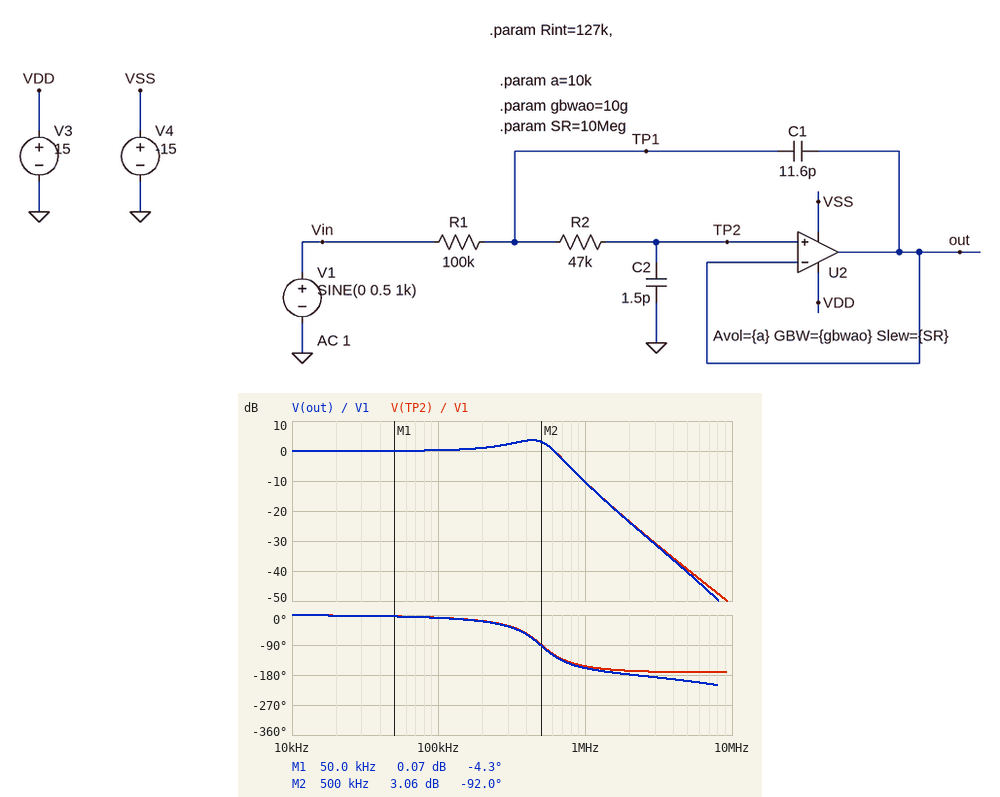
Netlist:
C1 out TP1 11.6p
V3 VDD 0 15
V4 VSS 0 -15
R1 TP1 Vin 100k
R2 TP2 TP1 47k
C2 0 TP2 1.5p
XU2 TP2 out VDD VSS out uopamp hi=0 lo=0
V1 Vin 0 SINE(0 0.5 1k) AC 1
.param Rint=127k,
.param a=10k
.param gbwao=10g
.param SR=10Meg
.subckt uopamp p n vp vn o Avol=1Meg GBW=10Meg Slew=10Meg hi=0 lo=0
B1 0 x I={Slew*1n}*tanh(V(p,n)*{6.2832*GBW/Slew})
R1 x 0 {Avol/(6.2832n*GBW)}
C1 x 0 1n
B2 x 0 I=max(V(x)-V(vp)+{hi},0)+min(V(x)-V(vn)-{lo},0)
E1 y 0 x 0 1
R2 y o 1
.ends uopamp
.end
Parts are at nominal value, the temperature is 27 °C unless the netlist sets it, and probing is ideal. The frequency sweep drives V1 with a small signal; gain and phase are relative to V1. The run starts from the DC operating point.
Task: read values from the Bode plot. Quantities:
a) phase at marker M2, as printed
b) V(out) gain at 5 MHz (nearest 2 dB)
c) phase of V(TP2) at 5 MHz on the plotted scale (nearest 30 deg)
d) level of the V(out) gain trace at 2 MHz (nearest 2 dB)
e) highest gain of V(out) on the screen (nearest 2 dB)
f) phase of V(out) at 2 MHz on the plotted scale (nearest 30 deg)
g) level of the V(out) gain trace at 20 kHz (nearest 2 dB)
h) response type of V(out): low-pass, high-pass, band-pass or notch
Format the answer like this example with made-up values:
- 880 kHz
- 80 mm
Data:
- -92.0 deg
- -40 dB
- -180 deg
- -24 dB
- 4 dB
- -180 deg
- 0 dB
- low-pass
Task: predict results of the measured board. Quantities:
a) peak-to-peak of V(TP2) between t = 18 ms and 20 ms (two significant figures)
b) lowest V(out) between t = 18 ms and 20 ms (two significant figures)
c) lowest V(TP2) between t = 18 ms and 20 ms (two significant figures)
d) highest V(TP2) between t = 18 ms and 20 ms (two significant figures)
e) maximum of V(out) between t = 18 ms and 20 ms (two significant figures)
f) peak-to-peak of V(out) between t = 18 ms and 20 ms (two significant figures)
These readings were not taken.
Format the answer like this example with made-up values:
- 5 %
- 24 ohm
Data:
- 1.0 V
- -500 mV
- -500 mV
- 500 mV
- 500 mV
- 1.0 V
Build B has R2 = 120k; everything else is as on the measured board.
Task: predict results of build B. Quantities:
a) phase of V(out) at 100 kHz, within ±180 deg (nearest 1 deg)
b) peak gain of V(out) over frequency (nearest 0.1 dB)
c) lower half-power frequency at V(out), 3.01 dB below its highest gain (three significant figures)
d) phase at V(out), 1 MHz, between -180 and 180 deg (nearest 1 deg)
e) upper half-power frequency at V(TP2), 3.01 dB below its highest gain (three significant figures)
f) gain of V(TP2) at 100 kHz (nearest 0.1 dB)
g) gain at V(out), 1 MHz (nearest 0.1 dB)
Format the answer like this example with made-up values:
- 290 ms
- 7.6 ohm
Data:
- -13 deg
- 3.7 dB
- 109 kHz
- -171 deg
- 396 kHz
- 0.6 dB
- -18.4 dB
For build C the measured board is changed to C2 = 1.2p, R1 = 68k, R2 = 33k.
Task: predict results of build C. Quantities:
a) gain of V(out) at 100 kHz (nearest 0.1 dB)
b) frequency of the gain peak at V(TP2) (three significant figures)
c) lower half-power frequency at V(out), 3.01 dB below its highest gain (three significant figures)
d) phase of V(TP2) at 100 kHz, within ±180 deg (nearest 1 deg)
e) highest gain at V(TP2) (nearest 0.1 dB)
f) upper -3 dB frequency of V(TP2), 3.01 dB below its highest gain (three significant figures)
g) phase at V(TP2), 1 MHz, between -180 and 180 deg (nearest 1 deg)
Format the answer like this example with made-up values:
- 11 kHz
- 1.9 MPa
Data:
- 0.1 dB
- 685 kHz
- 378 kHz
- -4 deg
- 4.9 dB
- 892 kHz
- -132 deg
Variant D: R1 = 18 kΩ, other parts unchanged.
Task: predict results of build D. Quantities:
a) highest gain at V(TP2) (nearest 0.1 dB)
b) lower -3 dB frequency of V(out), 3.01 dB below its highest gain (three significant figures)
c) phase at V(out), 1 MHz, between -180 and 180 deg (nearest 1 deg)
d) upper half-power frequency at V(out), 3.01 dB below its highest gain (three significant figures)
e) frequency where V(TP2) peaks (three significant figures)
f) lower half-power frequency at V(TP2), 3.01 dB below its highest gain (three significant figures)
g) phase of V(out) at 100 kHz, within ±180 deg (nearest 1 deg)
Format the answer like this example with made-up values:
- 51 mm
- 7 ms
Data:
- 3.2 dB
- 200 kHz
- -71 deg
- 1.40 MHz
- 1.00 MHz
- 222 kHz
- -4 deg
